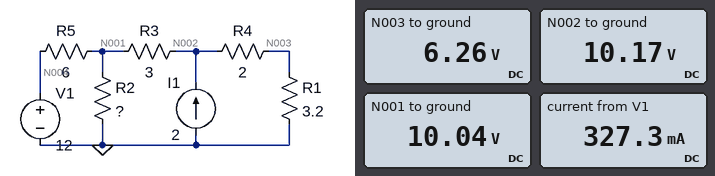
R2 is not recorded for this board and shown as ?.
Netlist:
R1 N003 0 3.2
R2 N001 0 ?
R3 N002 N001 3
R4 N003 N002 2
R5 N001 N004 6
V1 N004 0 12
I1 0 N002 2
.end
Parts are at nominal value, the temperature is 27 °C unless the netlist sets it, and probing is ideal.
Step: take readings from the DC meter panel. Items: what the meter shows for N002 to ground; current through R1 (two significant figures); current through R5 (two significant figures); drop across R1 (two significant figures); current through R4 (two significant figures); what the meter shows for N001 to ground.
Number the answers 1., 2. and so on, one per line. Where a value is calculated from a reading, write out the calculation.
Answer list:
1. 10.17 V
2. (6.26 V) / 3.2 Ω = 2.0 A
3. (12 V - 10.04 V) / 6 Ω = 330 mA
4. 6.26 V = 6.3 V
5. (10.17 V - 6.26 V) / 2 Ω = 2.0 A
6. 10.04 V
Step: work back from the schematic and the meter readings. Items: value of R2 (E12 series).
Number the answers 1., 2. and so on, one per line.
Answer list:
1. 27 Ω
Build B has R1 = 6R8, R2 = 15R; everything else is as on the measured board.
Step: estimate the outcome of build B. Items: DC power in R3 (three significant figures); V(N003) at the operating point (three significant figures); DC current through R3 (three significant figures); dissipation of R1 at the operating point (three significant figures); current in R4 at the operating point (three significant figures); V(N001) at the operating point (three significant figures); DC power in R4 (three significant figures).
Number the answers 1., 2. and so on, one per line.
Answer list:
1. 945 mW
2. 9.78 V
3. 561 mA
4. 14.1 W
5. 1.44 A
6. 11.0 V
7. 4.14 W
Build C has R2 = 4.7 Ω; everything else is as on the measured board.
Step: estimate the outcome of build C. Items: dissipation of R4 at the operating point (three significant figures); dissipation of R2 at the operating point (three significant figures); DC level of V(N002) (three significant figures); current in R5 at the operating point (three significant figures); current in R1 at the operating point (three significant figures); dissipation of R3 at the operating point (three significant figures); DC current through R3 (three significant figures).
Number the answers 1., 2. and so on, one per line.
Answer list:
1. 4.66 W
2. 9.04 W
3. 7.94 V
4. 914 mA
5. 1.53 A
6. 672 mW
7. 473 mA
